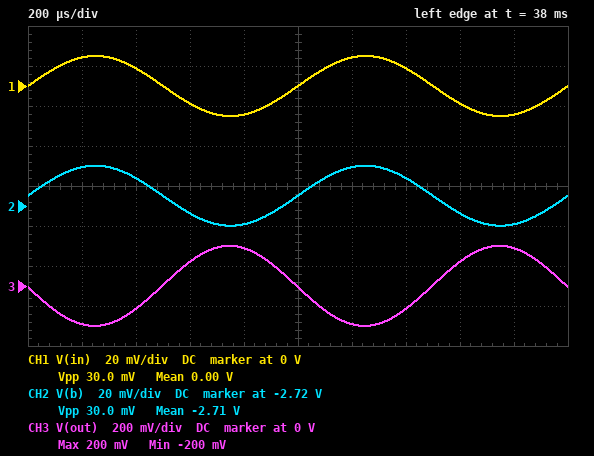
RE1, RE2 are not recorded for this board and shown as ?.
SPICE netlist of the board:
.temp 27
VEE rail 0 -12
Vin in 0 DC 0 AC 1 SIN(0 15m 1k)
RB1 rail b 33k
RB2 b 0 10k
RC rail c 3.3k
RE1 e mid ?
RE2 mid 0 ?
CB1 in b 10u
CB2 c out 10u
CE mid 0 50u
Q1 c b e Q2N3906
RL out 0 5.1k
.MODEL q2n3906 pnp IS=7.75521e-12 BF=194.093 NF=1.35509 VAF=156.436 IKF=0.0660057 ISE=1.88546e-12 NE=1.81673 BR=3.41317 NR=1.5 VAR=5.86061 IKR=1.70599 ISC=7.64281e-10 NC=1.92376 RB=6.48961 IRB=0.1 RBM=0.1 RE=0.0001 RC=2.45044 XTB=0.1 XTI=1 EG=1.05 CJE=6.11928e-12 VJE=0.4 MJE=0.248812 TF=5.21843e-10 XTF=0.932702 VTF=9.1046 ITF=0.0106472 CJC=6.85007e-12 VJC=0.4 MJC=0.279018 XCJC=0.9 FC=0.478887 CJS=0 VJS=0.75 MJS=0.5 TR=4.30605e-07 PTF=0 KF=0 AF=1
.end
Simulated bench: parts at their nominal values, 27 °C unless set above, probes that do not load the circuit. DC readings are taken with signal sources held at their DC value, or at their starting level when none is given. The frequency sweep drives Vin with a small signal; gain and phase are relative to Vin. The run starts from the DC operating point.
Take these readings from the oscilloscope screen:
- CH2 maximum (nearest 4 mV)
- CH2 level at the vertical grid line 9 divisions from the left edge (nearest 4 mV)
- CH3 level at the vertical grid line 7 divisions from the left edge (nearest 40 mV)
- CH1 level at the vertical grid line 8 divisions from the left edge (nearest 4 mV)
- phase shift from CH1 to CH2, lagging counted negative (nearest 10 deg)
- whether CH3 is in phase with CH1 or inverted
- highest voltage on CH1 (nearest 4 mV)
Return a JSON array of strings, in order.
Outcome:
["-2.700 V", "-2.728 V", "-120 mV", "-8 mV", "0 deg", "inverted", "16 mV"]
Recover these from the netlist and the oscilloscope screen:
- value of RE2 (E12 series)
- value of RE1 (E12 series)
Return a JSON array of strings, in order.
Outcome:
["1.5 kΩ", "120 Ω"]
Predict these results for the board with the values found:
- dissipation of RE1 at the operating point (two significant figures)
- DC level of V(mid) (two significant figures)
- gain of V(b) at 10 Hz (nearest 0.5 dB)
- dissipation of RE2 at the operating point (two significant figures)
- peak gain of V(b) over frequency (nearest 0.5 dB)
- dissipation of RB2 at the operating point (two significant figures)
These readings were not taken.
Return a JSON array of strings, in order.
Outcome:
["190 µW", "-1.9 V", "-0.5 dB", "2.4 mW", "0 dB", "740 µW"]
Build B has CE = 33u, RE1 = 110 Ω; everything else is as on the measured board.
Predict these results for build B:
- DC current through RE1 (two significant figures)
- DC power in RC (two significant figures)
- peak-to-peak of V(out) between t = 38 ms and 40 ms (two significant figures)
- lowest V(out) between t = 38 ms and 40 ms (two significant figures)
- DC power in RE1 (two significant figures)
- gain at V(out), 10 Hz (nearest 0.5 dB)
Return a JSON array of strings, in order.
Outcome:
["1.3 mA", "5.3 mW", "430 mV", "-210 mV", "180 µW", "11.0 dB"]
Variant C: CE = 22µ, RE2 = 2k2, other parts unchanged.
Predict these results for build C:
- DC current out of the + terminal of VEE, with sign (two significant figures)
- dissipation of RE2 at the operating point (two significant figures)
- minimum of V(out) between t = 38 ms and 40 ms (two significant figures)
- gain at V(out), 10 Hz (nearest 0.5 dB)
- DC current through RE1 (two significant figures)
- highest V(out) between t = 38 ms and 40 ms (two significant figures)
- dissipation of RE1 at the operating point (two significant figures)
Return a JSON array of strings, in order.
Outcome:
["-1.2 mA", "1.8 mW", "-180 mV", "8.0 dB", "900 µA", "190 mV", "97 µW"]
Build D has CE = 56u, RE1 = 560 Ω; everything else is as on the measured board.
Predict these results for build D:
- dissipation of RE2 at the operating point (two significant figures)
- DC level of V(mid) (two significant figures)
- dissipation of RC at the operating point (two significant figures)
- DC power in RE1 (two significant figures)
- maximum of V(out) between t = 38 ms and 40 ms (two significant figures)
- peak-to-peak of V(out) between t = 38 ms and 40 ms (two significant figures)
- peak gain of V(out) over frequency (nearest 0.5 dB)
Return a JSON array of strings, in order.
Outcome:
["1.5 mW", "-1.5 V", "3.3 mW", "570 µW", "50 mV", "100 mV", "10.5 dB"]
